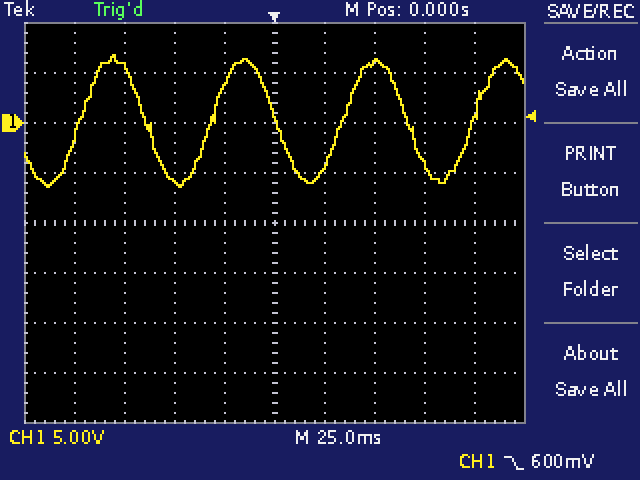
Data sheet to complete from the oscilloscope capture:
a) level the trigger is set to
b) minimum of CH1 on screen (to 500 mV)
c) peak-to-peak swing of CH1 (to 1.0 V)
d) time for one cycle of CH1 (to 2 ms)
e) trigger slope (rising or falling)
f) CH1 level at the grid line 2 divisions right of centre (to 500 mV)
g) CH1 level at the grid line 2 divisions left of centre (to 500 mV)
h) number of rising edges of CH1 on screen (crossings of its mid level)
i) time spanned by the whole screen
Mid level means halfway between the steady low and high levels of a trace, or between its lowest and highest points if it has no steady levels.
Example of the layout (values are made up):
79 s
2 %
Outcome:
600 mV
-6.5 V
13.0 V
66 ms
falling
6.0 V
-6.0 V
4
250 ms
